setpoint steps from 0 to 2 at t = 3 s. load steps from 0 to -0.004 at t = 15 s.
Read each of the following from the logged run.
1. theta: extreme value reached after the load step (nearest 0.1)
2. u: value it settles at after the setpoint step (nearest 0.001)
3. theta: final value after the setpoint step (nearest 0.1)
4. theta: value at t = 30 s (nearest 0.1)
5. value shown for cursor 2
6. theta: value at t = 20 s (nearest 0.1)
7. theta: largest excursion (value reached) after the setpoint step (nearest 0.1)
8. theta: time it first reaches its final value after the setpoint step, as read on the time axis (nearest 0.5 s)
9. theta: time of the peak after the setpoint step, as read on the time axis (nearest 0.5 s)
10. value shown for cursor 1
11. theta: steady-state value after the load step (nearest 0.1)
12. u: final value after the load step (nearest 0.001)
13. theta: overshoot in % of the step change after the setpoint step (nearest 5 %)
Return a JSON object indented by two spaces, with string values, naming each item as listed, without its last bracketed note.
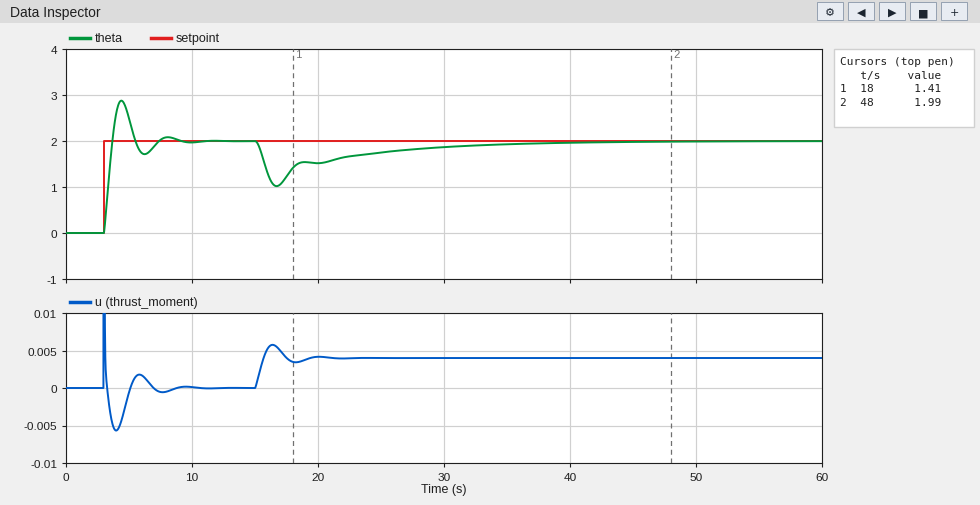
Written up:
{
  "theta: extreme value reached after the load step": "1.0",
  "u: value it settles at after the setpoint step": "0.000",
  "theta: final value after the setpoint step": "2.0",
  "theta: value at t = 30 s": "1.9",
  "value shown for cursor 2": "1.99",
  "theta: value at t = 20 s": "1.5",
  "theta: largest excursion (value reached) after the setpoint step": "2.9",
  "theta: time it first reaches its final value after the setpoint step, as read on the time axis": "3.5 s",
  "theta: time of the peak after the setpoint step, as read on the time axis": "4.5 s",
  "value shown for cursor 1": "1.41",
  "theta: steady-state value after the load step": "2.0",
  "u: final value after the load step": "0.004",
  "theta: overshoot in % of the step change after the setpoint step": "45 %"
}
